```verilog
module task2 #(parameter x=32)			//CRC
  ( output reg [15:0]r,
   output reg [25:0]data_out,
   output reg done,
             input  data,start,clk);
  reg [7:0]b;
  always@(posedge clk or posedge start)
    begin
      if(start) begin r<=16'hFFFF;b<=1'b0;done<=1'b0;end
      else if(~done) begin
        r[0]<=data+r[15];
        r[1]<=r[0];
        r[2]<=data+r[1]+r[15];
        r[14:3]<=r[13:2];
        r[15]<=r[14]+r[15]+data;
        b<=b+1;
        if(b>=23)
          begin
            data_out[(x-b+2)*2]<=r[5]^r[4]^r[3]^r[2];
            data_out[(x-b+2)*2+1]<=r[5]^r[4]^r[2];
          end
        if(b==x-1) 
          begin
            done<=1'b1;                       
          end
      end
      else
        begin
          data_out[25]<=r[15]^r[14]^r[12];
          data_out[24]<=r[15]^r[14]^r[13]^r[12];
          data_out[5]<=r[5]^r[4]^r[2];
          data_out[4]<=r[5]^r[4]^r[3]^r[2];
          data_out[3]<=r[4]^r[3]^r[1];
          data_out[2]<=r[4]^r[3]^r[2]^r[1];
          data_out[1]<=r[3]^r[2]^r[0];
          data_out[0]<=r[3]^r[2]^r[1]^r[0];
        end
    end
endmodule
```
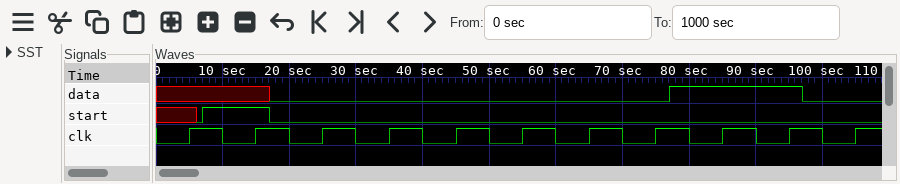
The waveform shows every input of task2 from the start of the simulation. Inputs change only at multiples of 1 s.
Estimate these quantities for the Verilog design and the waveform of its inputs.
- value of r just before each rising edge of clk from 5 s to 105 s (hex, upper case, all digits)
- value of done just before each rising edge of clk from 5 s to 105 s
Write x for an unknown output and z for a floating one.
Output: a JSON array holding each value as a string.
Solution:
["x, FFFF, FFFF, 7FFB, FFF6, 7FE9, FFD2, 7FA1, FF42, FE84, FD08", "x 0 0 0 0 0 0 0 0 0 0"]
